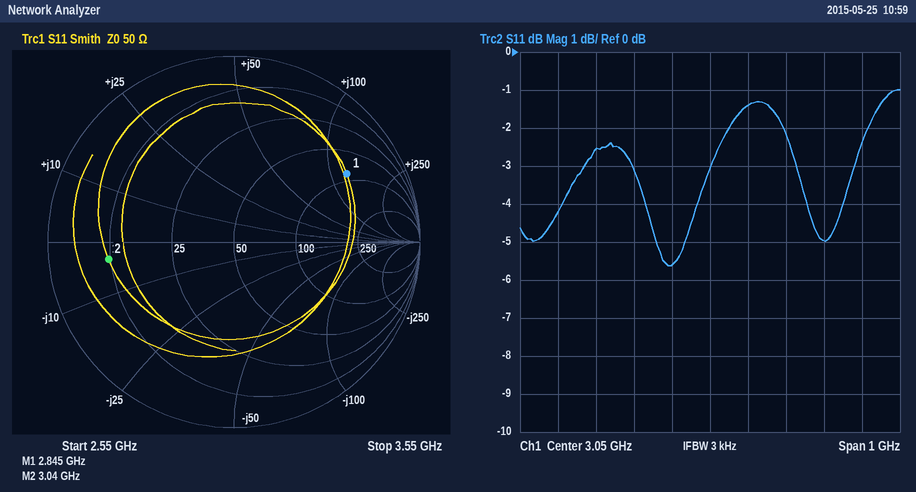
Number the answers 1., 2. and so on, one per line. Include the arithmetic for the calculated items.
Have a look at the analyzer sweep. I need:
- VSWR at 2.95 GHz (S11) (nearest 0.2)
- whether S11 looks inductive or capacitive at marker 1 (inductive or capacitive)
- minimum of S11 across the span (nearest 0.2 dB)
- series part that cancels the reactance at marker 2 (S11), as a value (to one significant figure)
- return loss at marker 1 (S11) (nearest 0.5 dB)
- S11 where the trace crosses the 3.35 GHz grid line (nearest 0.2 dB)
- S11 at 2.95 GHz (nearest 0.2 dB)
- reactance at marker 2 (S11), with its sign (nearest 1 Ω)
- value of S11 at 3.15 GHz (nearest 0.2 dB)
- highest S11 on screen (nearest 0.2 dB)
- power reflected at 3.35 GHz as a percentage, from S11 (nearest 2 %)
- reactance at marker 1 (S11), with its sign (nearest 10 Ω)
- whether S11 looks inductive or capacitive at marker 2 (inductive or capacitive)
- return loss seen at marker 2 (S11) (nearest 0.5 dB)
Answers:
1. |Γ| = 10^(-5.6/20) = 0.5248; VSWR = (1 + 0.5248)/(1 − 0.5248) ≈ 3.2
2. inductive
3. -5.6 dB
4. L = 3 Ω/(2π × 3.04 GHz) ≈ 157 pH, so 200 pH to one significant figure
5. 3.0 dB
6. -5.0 dB
7. -5.6 dB
8. -3 Ω
9. -1.4 dB
10. -1.0 dB
11. 10^(-5/10) ≈ 32 %
12. +130 Ω
13. capacitive
14. 3.5 dB
